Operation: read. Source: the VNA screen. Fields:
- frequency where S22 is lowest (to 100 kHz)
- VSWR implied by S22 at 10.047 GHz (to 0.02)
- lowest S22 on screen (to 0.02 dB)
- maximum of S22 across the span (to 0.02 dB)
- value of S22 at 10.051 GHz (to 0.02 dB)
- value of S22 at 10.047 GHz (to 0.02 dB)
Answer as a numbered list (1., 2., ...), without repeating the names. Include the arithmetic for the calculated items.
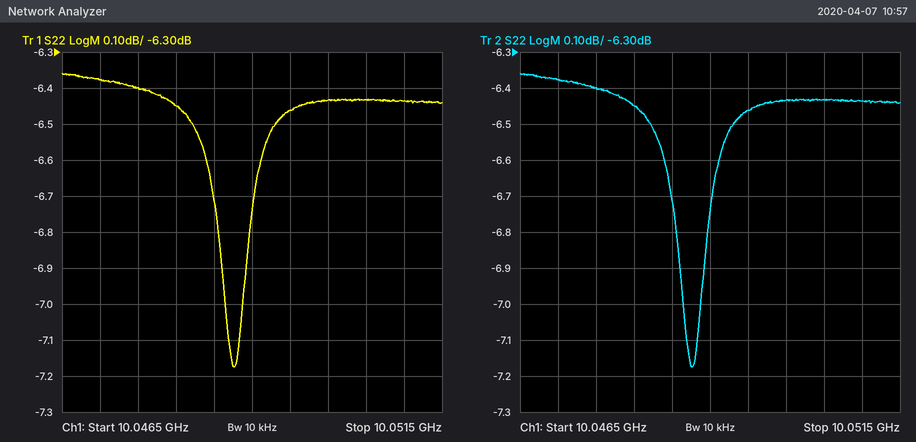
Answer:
1. 10.0488 GHz
2. |Γ| = 10^(-6.38/20) = 0.4797; VSWR = (1 + 0.4797)/(1 − 0.4797) ≈ 2.84
3. -7.18 dB
4. -6.36 dB
5. -6.44 dB
6. -6.38 dB
